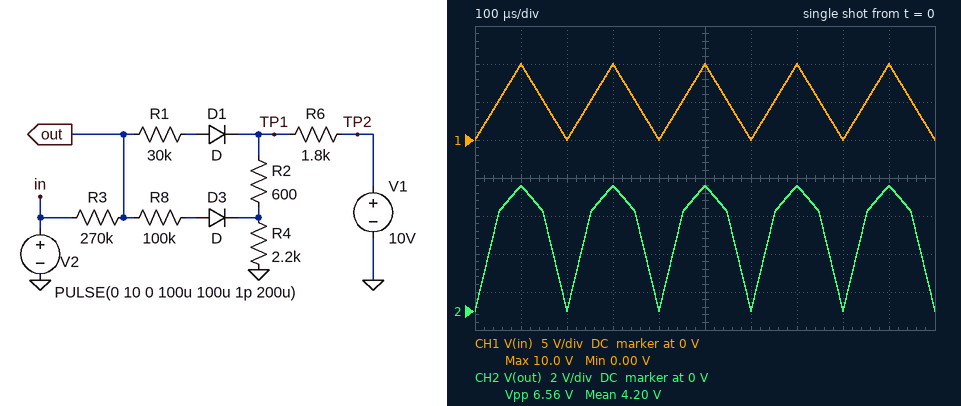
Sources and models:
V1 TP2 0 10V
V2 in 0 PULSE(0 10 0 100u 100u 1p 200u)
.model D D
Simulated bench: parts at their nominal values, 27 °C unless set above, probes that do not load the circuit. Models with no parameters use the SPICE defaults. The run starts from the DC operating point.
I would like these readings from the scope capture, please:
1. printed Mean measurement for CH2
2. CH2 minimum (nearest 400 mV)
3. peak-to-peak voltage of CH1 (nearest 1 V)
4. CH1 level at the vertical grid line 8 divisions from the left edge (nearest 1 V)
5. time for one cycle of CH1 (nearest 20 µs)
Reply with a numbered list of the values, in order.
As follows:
1. 4.20 V
2. 0 V
3. 10 V
4. 0 V
5. 200 µs
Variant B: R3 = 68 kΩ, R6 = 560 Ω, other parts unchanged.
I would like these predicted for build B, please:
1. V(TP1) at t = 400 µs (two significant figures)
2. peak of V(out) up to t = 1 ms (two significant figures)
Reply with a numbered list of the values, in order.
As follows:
1. 8.3 V
2. 8.8 V
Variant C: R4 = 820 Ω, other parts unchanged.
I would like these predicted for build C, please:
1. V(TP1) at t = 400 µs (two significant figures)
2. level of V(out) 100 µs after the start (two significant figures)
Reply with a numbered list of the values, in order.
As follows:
1. 4.4 V
2. 4.9 V
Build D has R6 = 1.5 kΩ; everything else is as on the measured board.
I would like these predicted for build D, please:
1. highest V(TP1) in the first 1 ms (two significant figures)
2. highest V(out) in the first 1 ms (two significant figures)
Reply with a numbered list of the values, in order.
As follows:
1. 6.5 V
2. 6.8 V
